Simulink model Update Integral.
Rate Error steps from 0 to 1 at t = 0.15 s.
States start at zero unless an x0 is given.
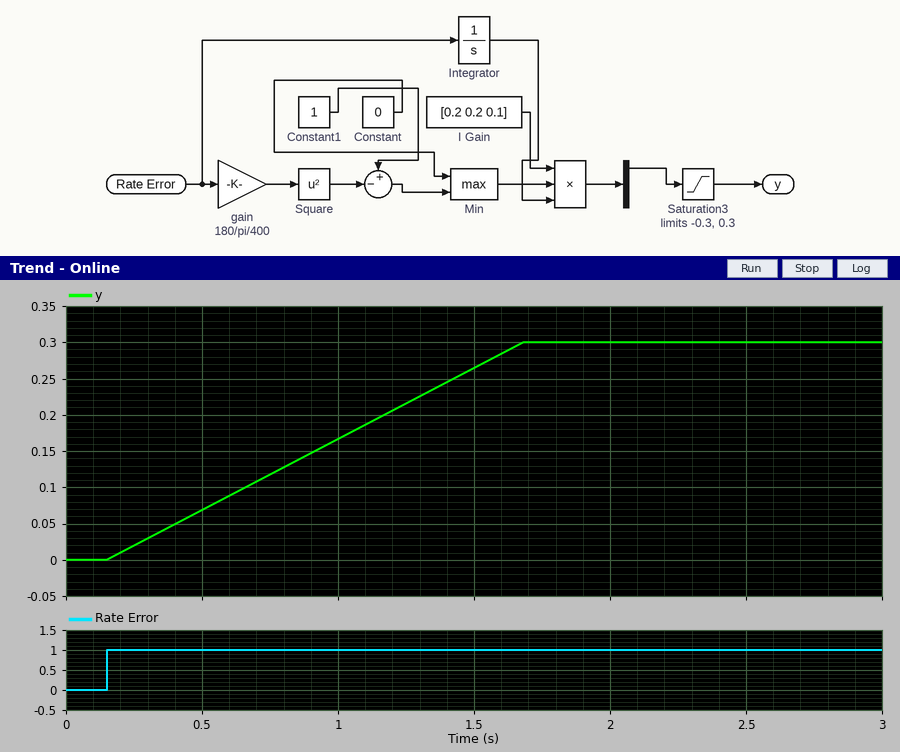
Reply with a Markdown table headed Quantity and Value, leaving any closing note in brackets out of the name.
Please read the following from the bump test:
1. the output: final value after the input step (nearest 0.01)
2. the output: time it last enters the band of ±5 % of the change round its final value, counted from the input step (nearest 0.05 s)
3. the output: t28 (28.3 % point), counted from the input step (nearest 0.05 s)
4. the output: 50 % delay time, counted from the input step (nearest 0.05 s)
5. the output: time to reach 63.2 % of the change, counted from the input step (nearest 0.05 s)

| Quantity | Value |
|---|---|
| the output: final value after the input step | 0.30 |
| the output: time it last enters the band of ±5 % of the change round its final value, counted from the input step | 1.45 s |
| the output: t28 (28.3 % point), counted from the input step | 0.45 s |
| the output: 50 % delay time, counted from the input step | 0.75 s |
| the output: time to reach 63.2 % of the change, counted from the input step | 0.95 s |
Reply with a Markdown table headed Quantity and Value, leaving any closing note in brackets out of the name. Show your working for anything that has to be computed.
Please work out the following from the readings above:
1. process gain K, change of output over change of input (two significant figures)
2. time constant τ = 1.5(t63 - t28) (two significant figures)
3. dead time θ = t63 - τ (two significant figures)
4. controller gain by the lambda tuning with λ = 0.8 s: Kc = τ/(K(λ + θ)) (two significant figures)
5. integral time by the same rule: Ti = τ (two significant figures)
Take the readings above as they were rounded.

| Quantity | Value |
|---|---|
| process gain K, change of output over change of input | (0.3 - 0) / 1 = 0.30 |
| time constant τ = 1.5(t63 - t28) | 1.5 × (0.95 - 0.45) = 0.75 s |
| dead time θ = t63 - τ | 0.95 - 0.75 = 0.20 s |
| controller gain by the lambda tuning with λ = 0.8 s: Kc = τ/(K(λ + θ)) | 0.75 / (0.3 × (0.8 + 0.2)) = 2.5 |
| integral time by the same rule: Ti = τ | 0.75 s |
